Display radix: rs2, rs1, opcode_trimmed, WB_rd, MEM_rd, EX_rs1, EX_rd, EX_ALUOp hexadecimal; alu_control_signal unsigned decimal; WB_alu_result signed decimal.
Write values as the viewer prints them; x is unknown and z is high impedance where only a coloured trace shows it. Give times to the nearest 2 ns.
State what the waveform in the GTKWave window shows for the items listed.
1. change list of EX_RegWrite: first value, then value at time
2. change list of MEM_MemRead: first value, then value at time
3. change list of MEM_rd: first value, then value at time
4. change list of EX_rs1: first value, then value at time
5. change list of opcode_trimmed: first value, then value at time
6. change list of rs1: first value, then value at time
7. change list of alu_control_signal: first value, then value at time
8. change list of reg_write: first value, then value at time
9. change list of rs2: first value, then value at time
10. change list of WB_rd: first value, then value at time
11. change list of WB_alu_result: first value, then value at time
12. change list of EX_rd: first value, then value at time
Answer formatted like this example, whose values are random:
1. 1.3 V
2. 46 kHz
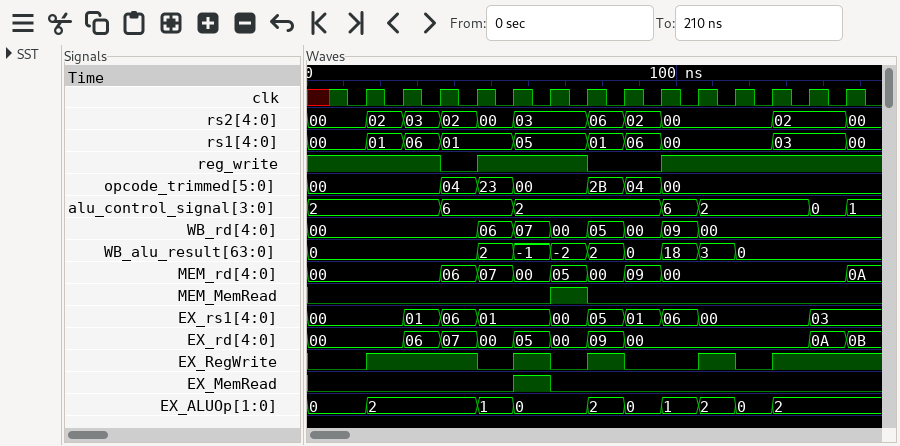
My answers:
1. 0, 1 at 16 ns, 0 at 46 ns, 1 at 56 ns, 0 at 66 ns, 1 at 76 ns, 0 at 86 ns, 1 at 106 ns, 0 at 116 ns, 1 at 126 ns
2. 0, 1 at 66 ns, 0 at 76 ns
3. 00, 06 at 36 ns, 07 at 46 ns, 00 at 56 ns, 05 at 66 ns, 00 at 76 ns, 09 at 86 ns, 00 at 96 ns, 0A at 146 ns
4. 00, 01 at 26 ns, 06 at 36 ns, 01 at 46 ns, 00 at 66 ns, 05 at 76 ns, 01 at 86 ns, 06 at 96 ns, 00 at 106 ns, 03 at 136 ns
5. 00, 04 at 36 ns, 23 at 46 ns, 00 at 56 ns, 2B at 76 ns, 04 at 86 ns, 00 at 96 ns
6. 00, 01 at 16 ns, 06 at 26 ns, 01 at 36 ns, 05 at 56 ns, 01 at 76 ns, 06 at 86 ns, 00 at 96 ns, 03 at 126 ns, 00 at 146 ns
7. 2, 6 at 36 ns, 2 at 56 ns, 6 at 96 ns, 2 at 106 ns, 0 at 136 ns, 1 at 146 ns
8. 1, 0 at 36 ns, 1 at 46 ns, 0 at 76 ns, 1 at 96 ns
9. 00, 02 at 16 ns, 03 at 26 ns, 02 at 36 ns, 00 at 46 ns, 03 at 56 ns, 06 at 76 ns, 02 at 86 ns, 00 at 96 ns, 02 at 126 ns, 00 at 146 ns
10. 00, 06 at 46 ns, 07 at 56 ns, 00 at 66 ns, 05 at 76 ns, 00 at 86 ns, 09 at 96 ns, 00 at 106 ns
11. 0, 2 at 46 ns, -1 at 56 ns, -2 at 66 ns, 2 at 76 ns, 0 at 86 ns, 18 at 96 ns, 3 at 106 ns, 0 at 116 ns
12. 00, 06 at 26 ns, 07 at 36 ns, 00 at 46 ns, 05 at 56 ns, 00 at 66 ns, 09 at 76 ns, 00 at 86 ns, 0A at 136 ns, 0B at 146 ns
